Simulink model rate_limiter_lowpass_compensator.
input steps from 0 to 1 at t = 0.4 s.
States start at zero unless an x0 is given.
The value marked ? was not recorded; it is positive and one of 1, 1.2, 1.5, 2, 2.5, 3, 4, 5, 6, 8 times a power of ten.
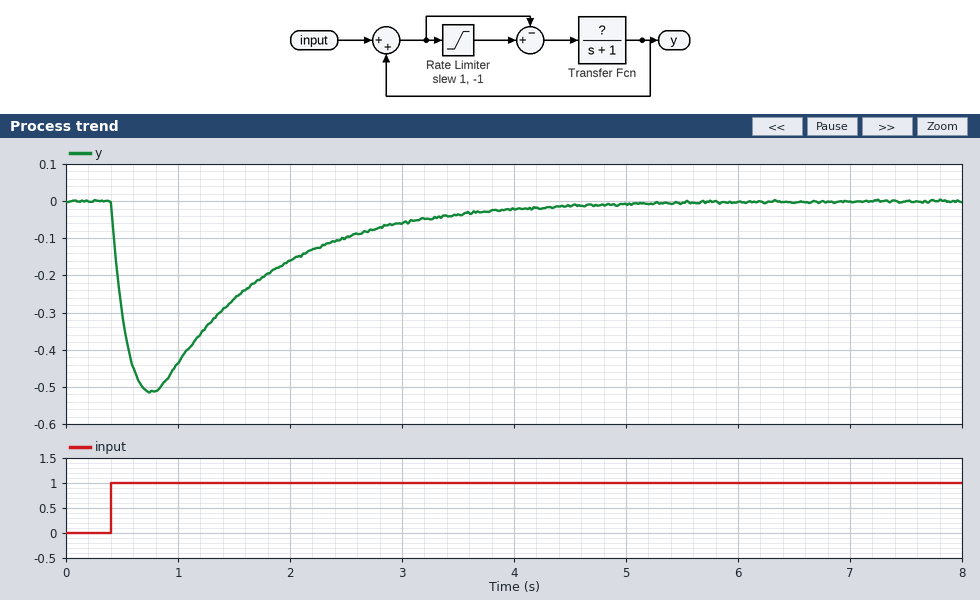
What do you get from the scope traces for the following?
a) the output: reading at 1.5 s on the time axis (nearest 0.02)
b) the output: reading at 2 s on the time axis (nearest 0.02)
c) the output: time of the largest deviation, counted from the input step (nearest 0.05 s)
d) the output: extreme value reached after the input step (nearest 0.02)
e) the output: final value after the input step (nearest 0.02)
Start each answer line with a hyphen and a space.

- -0.26
- -0.16
- 0.35 s
- -0.52
- 0.00
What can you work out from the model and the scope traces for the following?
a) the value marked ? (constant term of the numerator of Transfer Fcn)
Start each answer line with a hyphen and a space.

- 4
